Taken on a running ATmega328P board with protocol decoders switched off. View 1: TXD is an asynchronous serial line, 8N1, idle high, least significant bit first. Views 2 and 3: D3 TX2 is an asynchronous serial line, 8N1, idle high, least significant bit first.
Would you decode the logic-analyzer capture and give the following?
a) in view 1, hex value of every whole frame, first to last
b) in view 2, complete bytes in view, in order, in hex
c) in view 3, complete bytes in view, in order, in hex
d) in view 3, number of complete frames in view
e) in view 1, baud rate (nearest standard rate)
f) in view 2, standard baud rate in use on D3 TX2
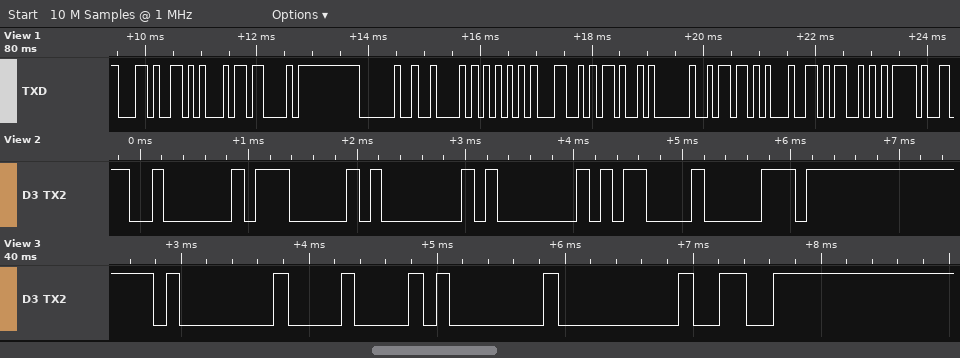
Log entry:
2C 45 43 20 42 55 4C 4B 20 5B 64 53 2F
02 07 01 01 0D 70
0x01 0x08 0x01 0x00 0xE6
5
9600 baud
9600 baud
